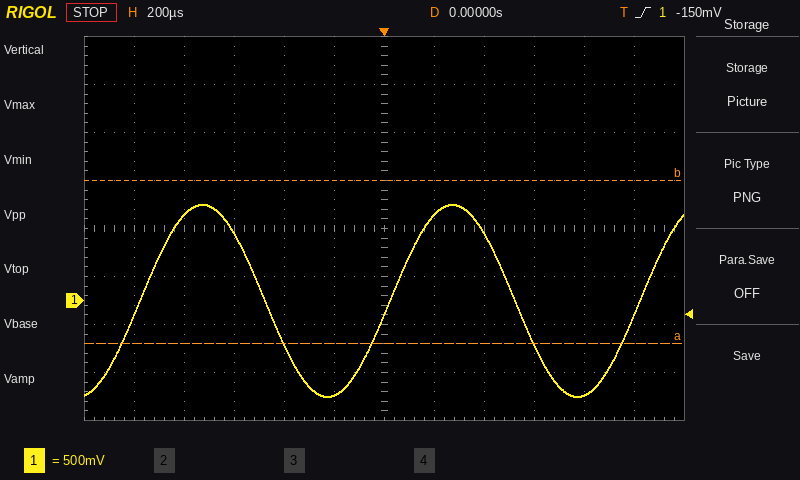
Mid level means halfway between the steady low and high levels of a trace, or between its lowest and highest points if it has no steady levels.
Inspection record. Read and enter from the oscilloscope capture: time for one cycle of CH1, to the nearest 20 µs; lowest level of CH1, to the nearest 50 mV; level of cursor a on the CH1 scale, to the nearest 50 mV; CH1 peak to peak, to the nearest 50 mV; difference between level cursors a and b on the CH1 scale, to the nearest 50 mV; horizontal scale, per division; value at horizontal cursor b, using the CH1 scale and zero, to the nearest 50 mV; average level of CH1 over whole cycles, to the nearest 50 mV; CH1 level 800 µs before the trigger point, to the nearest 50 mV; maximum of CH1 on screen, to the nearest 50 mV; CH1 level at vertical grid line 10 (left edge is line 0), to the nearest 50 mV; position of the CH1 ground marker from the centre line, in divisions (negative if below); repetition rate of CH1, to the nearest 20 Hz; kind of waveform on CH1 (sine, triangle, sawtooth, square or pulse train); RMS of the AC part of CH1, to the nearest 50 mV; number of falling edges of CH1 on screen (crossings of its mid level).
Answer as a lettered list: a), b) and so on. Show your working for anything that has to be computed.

a) 1.00 ms
b) -1.00 V
c) -450 mV
d) 1.00 V − (-1.00 V) = 2.00 V
e) 1.70 V
f) 200 µs
g) 1.25 V
h) (1.00 V + (-1.00 V)) / 2 ≈ 0 mV
i) 900 mV
j) 1.00 V
k) -1.00 V
l) -1.5 div
m) 1 / 1.00 ms ≈ 1.00 kHz
n) sine
o) 2.00 V / (2√2) ≈ 707 mV, so 700 mV to the nearest 50 mV
p) 2
